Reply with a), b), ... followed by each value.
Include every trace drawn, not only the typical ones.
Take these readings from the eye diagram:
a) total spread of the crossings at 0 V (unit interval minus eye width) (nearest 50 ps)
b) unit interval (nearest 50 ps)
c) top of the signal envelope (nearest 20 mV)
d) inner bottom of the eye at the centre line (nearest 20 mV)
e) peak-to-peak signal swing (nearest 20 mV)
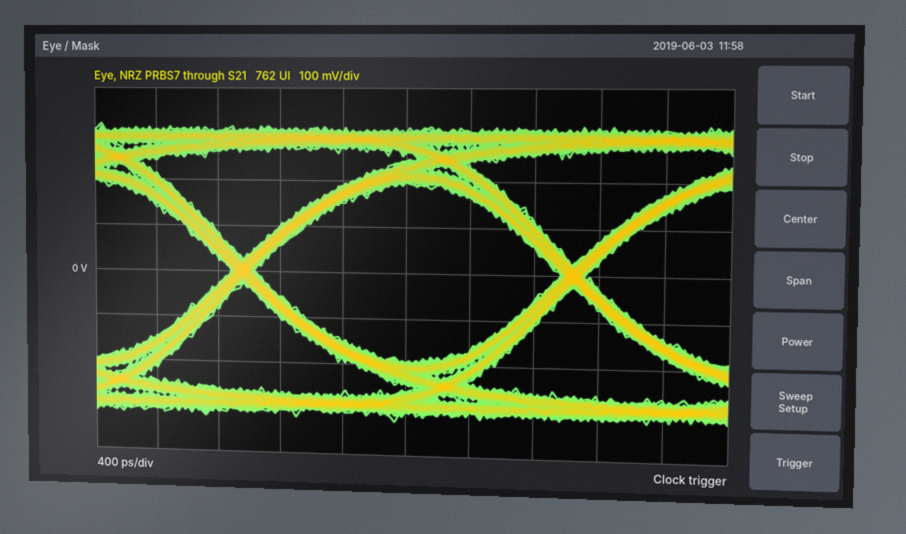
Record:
a) 150 ps
b) 2.10 ns
c) 320 mV
d) -200 mV
e) 640 mV
